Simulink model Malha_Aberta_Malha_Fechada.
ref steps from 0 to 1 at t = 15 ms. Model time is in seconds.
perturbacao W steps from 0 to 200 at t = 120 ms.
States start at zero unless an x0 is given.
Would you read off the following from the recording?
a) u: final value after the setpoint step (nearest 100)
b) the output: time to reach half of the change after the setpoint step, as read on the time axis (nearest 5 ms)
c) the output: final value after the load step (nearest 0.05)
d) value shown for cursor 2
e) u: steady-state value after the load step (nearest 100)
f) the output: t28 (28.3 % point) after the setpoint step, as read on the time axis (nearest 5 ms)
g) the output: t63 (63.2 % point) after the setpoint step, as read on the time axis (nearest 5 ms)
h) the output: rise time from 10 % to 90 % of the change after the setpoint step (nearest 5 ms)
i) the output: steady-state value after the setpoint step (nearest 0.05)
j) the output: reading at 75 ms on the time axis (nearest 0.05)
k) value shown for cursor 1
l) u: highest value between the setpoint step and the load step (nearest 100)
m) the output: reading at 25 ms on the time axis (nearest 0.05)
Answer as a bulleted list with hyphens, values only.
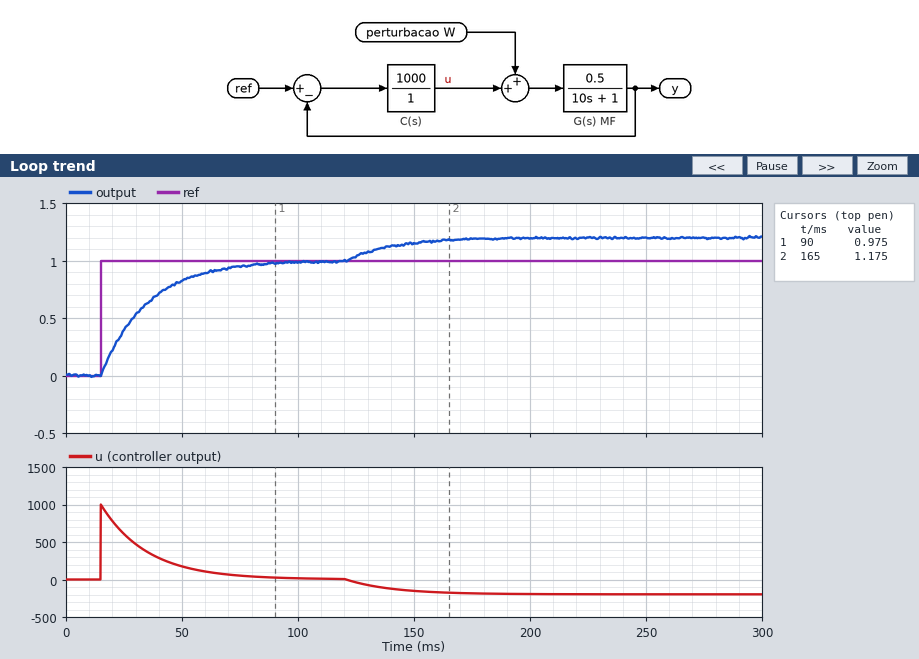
- 0
- 30 ms
- 1.20
- 1.175
- -200
- 20 ms
- 35 ms
- 45 ms
- 1.00
- 0.95
- 0.975
- 1000
- 0.40
